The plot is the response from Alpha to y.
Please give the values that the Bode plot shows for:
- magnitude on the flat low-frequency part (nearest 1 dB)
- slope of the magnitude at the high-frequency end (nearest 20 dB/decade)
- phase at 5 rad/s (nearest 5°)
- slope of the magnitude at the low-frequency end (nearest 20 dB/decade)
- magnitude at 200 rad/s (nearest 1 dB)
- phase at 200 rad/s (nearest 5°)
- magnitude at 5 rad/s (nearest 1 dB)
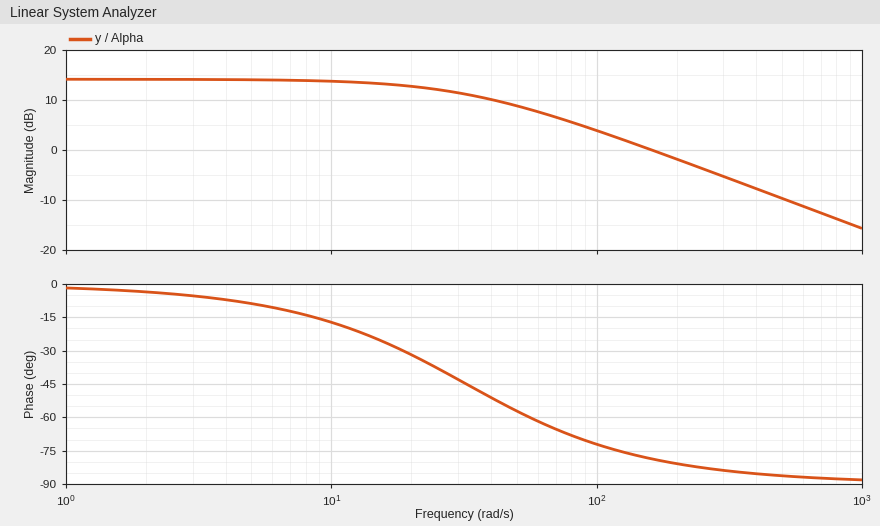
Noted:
14 dB
-20 dB/decade
-10°
0 dB/decade
-2 dB
-80°
14 dB
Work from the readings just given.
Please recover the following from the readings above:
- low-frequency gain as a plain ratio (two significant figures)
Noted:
5.0
